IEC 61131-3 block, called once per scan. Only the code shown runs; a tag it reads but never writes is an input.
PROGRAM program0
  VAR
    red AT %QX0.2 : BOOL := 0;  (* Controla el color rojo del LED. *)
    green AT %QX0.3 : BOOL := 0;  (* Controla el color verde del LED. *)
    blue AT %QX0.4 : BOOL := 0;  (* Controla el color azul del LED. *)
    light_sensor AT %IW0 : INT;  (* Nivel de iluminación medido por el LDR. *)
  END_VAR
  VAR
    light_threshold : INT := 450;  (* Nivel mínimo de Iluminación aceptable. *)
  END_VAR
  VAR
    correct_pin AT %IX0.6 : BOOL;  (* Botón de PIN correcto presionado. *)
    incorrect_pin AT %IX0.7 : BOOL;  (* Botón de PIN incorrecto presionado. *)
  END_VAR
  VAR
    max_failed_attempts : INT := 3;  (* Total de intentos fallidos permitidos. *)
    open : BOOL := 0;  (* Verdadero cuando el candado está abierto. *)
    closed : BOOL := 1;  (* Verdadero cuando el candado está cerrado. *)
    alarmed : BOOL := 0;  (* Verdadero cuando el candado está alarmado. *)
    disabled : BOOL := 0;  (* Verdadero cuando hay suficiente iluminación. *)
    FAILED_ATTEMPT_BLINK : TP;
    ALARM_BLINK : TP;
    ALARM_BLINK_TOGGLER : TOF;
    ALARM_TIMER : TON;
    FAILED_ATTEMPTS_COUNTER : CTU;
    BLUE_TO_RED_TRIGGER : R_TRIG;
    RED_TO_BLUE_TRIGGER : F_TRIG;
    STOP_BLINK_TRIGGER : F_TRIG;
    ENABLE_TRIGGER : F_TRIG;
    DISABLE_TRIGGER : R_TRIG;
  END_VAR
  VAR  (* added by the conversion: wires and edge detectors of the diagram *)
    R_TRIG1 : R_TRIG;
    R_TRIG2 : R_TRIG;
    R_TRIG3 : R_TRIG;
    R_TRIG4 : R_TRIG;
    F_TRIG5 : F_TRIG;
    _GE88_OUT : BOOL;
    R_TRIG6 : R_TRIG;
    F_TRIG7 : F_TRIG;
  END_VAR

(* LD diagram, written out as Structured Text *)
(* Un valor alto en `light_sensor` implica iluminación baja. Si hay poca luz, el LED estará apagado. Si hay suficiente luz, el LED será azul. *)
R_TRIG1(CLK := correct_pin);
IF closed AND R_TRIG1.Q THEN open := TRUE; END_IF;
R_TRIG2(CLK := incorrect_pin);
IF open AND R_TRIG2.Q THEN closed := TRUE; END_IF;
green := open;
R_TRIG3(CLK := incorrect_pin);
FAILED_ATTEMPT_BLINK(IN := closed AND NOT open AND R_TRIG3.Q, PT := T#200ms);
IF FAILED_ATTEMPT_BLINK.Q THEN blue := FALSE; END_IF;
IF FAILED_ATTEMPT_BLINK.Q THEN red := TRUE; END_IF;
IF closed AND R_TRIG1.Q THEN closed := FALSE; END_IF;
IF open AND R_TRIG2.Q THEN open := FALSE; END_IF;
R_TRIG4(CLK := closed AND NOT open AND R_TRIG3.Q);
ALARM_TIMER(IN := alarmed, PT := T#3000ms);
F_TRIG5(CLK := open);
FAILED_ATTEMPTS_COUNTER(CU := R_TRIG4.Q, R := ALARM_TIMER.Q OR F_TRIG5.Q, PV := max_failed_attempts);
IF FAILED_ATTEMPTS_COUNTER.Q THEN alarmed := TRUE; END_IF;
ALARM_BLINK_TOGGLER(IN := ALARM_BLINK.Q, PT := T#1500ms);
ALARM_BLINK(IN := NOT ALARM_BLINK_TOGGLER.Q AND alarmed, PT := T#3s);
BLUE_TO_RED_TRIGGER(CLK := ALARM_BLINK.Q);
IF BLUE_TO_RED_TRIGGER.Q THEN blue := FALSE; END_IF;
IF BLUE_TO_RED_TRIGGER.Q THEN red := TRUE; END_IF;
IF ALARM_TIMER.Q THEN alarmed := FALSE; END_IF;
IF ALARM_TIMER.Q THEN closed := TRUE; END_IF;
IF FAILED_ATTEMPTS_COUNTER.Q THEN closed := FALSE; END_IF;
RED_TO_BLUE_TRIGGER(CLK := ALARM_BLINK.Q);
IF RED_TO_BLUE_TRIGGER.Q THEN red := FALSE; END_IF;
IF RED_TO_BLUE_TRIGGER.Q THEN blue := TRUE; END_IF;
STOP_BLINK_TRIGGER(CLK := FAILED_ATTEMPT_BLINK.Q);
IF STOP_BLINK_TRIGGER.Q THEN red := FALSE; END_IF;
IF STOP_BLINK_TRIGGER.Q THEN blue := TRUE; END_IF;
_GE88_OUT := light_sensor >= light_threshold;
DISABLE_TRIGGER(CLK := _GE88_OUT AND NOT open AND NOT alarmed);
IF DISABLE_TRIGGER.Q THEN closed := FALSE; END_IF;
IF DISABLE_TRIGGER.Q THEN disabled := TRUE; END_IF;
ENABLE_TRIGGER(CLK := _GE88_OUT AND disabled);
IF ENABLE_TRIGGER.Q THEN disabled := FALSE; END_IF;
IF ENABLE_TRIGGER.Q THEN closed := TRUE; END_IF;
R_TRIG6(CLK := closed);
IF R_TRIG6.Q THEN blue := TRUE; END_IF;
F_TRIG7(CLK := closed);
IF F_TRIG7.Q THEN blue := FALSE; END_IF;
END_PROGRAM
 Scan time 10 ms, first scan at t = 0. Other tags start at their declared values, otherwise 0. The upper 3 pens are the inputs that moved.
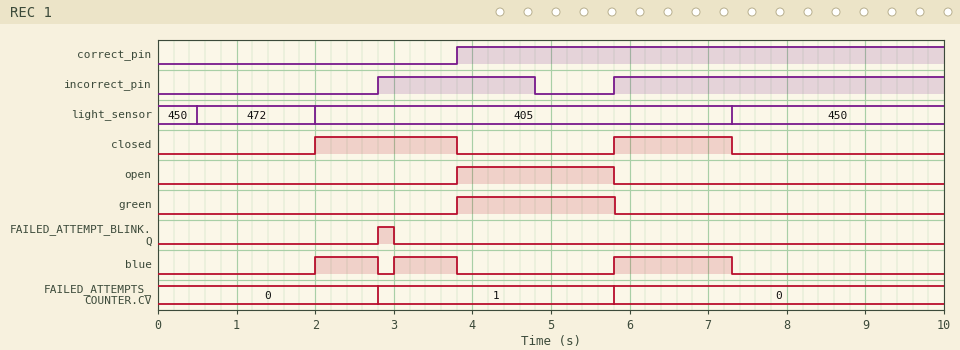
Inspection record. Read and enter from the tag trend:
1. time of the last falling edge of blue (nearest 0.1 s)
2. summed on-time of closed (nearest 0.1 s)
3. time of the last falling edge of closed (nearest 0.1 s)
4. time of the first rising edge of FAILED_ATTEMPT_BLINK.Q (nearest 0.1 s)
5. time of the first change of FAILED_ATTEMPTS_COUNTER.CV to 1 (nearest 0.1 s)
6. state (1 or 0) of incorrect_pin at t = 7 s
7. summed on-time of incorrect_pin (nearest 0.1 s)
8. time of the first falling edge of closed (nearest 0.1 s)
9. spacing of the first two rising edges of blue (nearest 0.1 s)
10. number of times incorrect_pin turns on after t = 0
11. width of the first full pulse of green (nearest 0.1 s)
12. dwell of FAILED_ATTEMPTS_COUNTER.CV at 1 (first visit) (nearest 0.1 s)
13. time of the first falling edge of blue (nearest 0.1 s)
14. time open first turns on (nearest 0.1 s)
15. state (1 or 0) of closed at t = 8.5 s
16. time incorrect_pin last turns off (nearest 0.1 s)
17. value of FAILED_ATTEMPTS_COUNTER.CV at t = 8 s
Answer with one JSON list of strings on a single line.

["7.3 s", "3.3 s", "7.3 s", "2.8 s", "2.8 s", "1", "6.2 s", "3.8 s", "1.0 s", "2", "2.0 s", "3.0 s", "2.8 s", "3.8 s", "0", "4.8 s", "0"]
